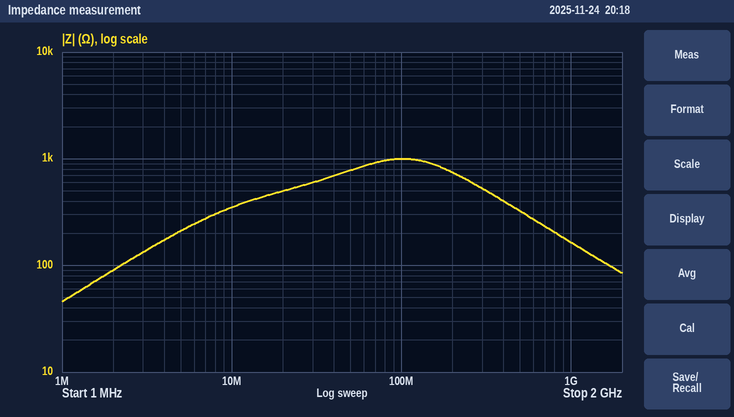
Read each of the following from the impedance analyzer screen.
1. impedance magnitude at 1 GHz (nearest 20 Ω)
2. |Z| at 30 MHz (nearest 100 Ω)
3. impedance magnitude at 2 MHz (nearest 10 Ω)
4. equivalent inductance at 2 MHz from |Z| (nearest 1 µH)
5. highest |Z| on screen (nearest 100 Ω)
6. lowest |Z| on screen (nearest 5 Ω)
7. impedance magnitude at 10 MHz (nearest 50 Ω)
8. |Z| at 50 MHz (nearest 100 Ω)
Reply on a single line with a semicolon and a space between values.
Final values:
160 Ω; 600 Ω; 90 Ω; 7 µH; 1.0 kΩ; 45 Ω; 350 Ω; 800 Ω
